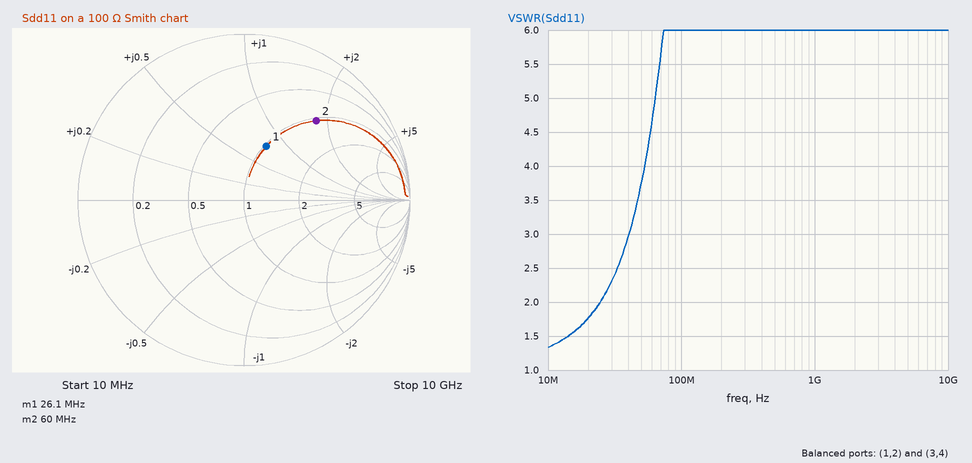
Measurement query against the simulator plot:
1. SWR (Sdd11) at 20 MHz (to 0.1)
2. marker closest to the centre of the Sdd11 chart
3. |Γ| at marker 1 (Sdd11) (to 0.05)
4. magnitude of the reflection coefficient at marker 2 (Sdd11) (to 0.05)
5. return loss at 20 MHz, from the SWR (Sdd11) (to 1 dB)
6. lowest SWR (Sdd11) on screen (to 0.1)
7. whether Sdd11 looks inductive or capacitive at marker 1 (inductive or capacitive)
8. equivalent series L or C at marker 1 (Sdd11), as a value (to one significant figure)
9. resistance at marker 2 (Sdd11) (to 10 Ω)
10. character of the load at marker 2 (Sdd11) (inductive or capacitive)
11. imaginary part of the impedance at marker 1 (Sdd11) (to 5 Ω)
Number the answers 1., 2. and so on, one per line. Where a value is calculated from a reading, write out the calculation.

1. 1.8
2. marker 1
3. 0.35
4. 0.65
5. −20 log10((1.8 − 1)/(1.8 + 1)) ≈ 11 dB
6. 1.3
7. inductive
8. L = 75 Ω/(2π × 26.1 MHz) ≈ 457 nH, so 500 nH to one significant figure
9. 110 Ω
10. inductive
11. +75 Ω
